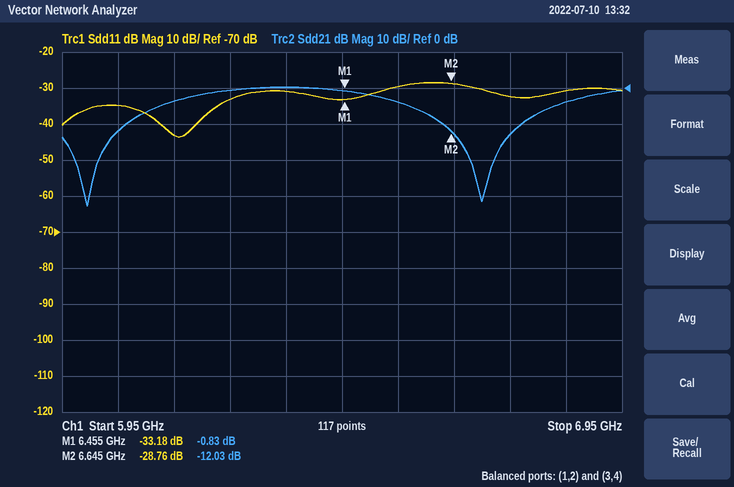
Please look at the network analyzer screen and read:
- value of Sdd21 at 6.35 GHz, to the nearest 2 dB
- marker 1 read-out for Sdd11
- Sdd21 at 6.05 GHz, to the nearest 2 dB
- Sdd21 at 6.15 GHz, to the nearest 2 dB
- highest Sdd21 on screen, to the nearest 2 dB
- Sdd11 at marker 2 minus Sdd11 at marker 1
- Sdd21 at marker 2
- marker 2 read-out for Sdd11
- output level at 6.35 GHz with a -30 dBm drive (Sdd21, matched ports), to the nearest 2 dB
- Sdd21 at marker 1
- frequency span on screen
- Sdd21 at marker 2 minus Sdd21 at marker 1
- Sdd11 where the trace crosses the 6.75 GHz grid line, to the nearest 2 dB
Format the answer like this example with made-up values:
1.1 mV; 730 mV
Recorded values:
0 dB; -33.18 dB; -12 dB; -4 dB; 0 dB; 4.42 dB; -12.03 dB; -28.76 dB; -30 dBm; -0.83 dB; 1 GHz; -11.20 dB; -32 dB
